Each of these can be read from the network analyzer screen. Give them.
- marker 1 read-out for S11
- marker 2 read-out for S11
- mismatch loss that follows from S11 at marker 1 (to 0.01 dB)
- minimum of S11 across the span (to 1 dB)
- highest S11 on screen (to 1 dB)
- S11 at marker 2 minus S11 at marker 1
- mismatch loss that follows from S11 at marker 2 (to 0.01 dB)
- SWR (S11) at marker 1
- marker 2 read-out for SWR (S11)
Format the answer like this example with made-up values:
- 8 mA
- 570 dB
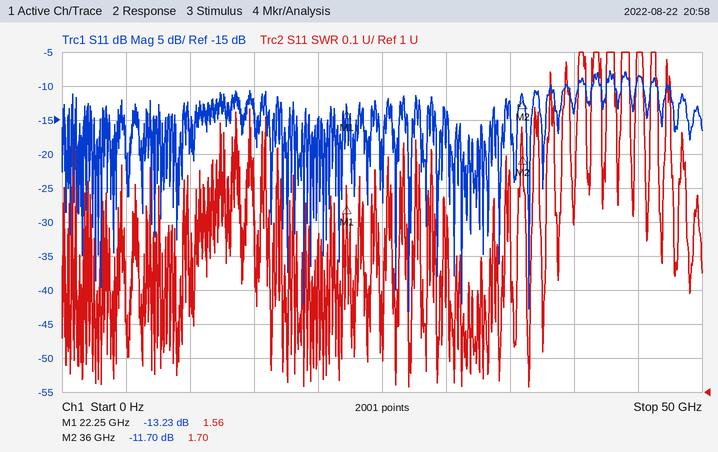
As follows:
- -13.23 dB
- -11.70 dB
- 0.21 dB
- -43 dB
- -8 dB
- 1.53 dB
- 0.30 dB
- 1.56
- 1.70
